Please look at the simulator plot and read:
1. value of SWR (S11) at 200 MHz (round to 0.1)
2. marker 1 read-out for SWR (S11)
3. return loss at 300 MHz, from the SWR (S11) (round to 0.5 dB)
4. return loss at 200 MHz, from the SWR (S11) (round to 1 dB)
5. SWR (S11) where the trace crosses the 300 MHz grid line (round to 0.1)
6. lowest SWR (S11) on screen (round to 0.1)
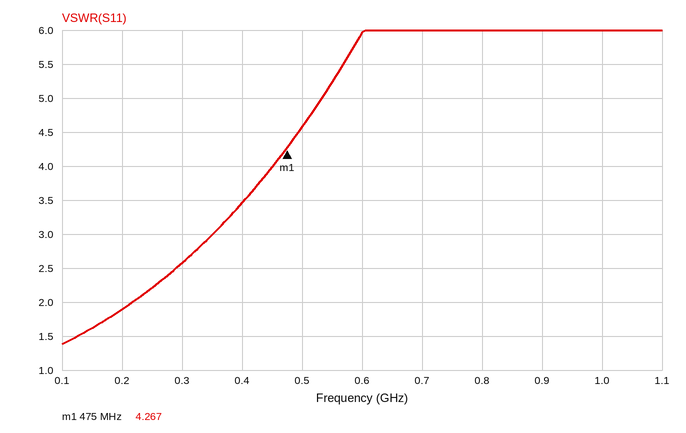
1.9
4.267
7.0 dB
10 dB
2.6
1.4
